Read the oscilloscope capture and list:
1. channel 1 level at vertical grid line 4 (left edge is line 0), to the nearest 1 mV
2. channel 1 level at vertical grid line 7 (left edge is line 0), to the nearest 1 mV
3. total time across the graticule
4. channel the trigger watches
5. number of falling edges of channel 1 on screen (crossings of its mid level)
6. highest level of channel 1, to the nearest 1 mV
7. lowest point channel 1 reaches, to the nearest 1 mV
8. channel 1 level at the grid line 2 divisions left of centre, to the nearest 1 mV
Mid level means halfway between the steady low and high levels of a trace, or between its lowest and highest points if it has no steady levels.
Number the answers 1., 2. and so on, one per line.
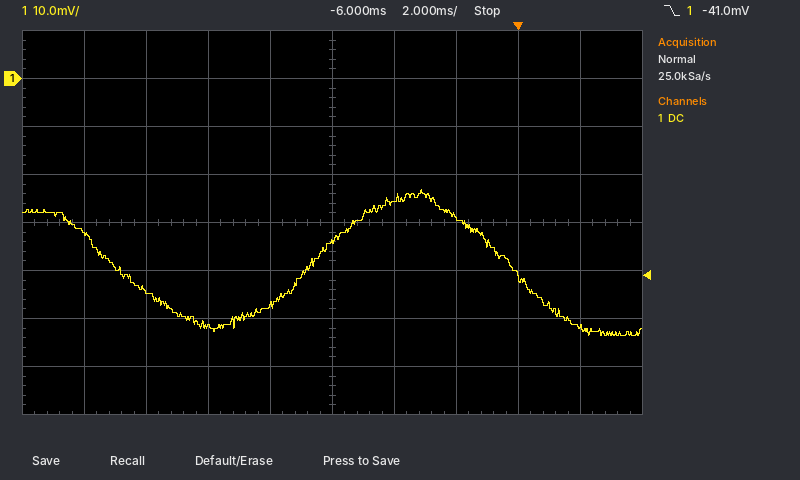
1. -47 mV
2. -29 mV
3. 20 ms
4. channel 1
5. 2
6. -23 mV
7. -54 mV
8. -52 mV
